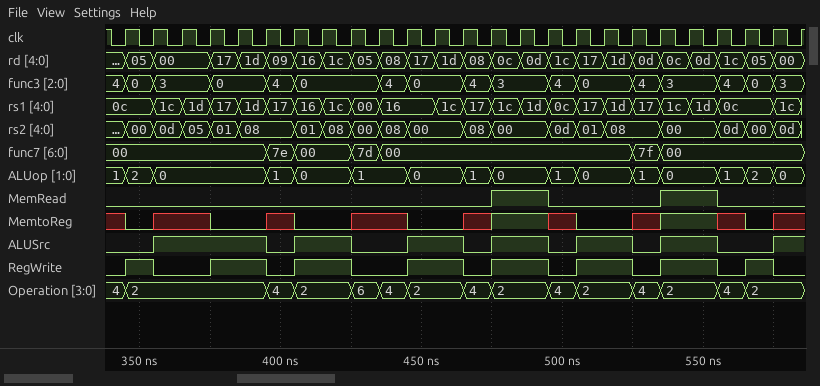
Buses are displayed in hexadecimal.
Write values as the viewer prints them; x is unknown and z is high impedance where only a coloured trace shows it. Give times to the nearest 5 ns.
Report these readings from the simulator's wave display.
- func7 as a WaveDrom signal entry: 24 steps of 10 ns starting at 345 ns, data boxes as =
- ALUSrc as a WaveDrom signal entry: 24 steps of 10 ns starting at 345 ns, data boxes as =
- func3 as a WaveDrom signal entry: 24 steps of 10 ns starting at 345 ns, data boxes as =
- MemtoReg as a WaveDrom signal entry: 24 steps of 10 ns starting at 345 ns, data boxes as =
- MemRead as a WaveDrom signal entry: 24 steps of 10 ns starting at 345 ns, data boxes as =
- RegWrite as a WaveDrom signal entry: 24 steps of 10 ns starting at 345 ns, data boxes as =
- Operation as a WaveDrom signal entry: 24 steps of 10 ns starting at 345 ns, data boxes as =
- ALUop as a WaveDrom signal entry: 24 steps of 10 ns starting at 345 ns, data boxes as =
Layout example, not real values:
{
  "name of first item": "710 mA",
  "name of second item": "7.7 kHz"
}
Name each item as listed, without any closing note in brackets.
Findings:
{
  "func7 as a WaveDrom signal entry: 24 steps of 10 ns starting at 345 ns, data boxes as =": "{name: 'func7', wave: '=....==.==........==....', data: '00 7e 00 7d 00 7f 00'}",
  "ALUSrc as a WaveDrom signal entry: 24 steps of 10 ns starting at 345 ns, data boxes as =": "{name: 'ALUSrc', wave: '01...01.0.1.01.01.01.0.1'}",
  "func3 as a WaveDrom signal entry: 24 steps of 10 ns starting at 345 ns, data boxes as =": "{name: 'func3', wave: '==.=.==..==.==.==.==.===', data: '0 3 0 4 0 4 0 4 3 4 0 4 3 4 0 3'}",
  "MemtoReg as a WaveDrom signal entry: 24 steps of 10 ns starting at 345 ns, data boxes as =": "{name: 'MemtoReg', wave: '0x.0.x0.x.0.x1.x0.x1.x0x'}",
  "MemRead as a WaveDrom signal entry: 24 steps of 10 ns starting at 345 ns, data boxes as =": "{name: 'MemRead', wave: '0............1.0...1.0..'}",
  "RegWrite as a WaveDrom signal entry: 24 steps of 10 ns starting at 345 ns, data boxes as =": "{name: 'RegWrite', wave: '10.1.01.0.1.01.01.01.010'}",
  "Operation as a WaveDrom signal entry: 24 steps of 10 ns starting at 345 ns, data boxes as =": "{name: 'Operation', wave: '=....==.===.==.==.==.==.', data: '2 4 2 6 4 2 4 2 4 2 4 2 4 2'}",
  "ALUop as a WaveDrom signal entry: 24 steps of 10 ns starting at 345 ns, data boxes as =": "{name: 'ALUop', wave: '==...==.=.=.==.==.==.===', data: '2 0 1 0 1 0 1 0 1 0 1 0 1 2 0'}"
}
